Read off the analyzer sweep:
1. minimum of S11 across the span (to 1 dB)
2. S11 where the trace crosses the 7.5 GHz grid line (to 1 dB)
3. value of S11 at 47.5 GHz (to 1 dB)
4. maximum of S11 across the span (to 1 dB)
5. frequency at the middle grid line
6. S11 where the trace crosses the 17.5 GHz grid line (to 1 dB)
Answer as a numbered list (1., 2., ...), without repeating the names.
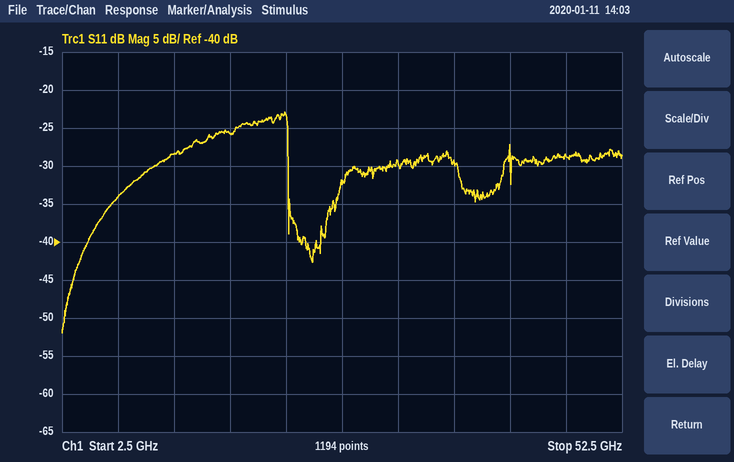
1. -52 dB
2. -34 dB
3. -29 dB
4. -23 dB
5. 27.5 GHz
6. -26 dB
